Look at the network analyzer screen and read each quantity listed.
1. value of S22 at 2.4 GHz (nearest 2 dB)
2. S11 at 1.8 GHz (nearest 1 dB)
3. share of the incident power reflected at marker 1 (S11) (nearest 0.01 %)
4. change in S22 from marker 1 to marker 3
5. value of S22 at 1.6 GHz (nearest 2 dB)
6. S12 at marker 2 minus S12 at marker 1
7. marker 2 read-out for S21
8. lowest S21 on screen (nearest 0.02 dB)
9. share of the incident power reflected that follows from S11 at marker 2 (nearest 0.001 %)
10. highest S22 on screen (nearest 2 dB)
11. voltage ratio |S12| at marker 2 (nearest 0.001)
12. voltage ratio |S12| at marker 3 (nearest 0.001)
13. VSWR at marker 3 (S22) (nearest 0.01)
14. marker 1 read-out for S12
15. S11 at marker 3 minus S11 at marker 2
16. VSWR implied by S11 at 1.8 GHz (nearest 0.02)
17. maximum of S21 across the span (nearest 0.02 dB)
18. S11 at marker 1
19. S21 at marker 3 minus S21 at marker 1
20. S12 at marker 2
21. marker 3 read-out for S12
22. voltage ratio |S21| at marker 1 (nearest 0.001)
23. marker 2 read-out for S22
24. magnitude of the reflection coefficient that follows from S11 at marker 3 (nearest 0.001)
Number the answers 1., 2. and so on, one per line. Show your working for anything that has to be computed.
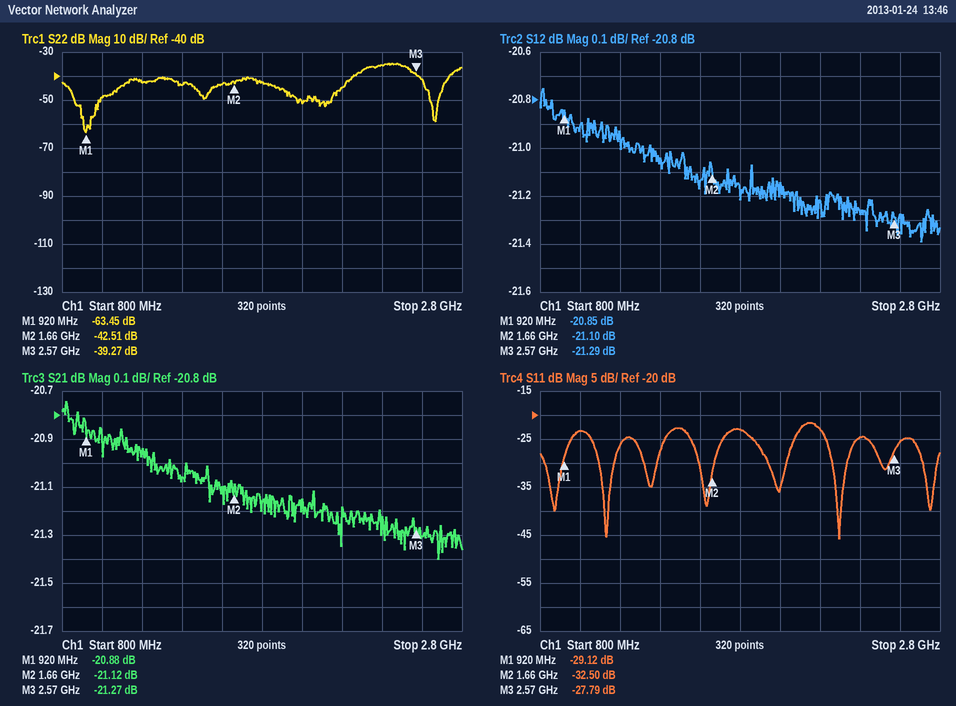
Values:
1. -36 dB
2. -23 dB
3. 10^(-29.12/10) ≈ 0.12 %
4. -39.27 − (-63.45) = 24.18 dB
5. -44 dB
6. -21.1 − (-20.85) = -0.25 dB
7. -21.12 dB
8. -21.40 dB
9. 10^(-32.5/10) ≈ 0.056 %
10. -34 dB
11. 10^(-21.1/20) ≈ 0.088
12. 10^(-21.29/20) ≈ 0.086
13. (1 + 0.0109)/(1 − 0.0109) ≈ 1.02
14. -20.85 dB
15. -27.79 − (-32.5) = 4.71 dB
16. |Γ| = 10^(-23/20) = 0.0708; VSWR = (1 + 0.0708)/(1 − 0.0708) ≈ 1.15, so 1.16 to the nearest 0.02
17. -20.74 dB
18. -29.12 dB
19. -21.27 − (-20.88) = -0.39 dB
20. -21.10 dB
21. -21.29 dB
22. 10^(-20.88/20) ≈ 0.090
23. -42.51 dB
24. 10^(-27.79/20) ≈ 0.041
